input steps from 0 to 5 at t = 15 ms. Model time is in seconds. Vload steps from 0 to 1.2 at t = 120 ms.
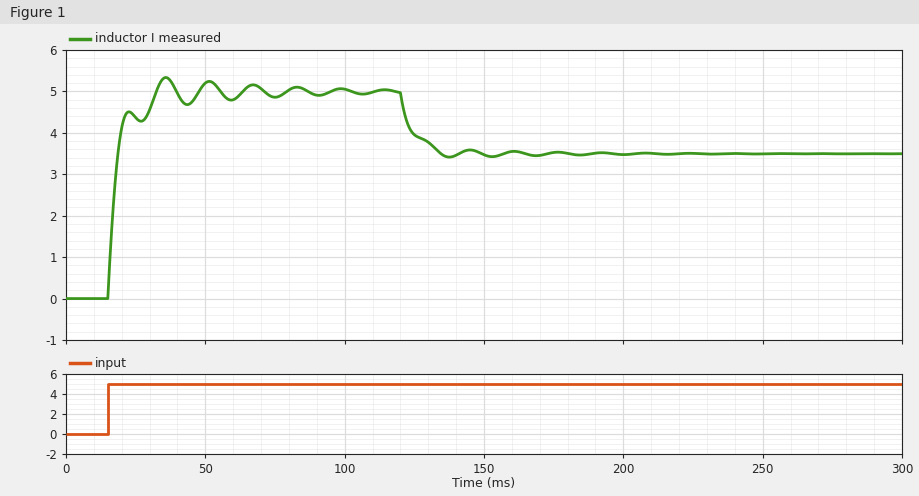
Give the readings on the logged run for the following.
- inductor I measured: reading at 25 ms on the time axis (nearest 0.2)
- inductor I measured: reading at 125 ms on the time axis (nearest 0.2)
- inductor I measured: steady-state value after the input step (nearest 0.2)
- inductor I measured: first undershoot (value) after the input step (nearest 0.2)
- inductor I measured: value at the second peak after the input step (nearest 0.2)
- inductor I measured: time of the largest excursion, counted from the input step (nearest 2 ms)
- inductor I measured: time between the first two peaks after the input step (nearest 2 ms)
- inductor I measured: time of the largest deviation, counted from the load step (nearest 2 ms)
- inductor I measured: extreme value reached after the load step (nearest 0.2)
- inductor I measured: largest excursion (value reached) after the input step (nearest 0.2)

4.4
4.0
5.0
4.6
5.2
20 ms
16 ms
18 ms
3.4
5.4
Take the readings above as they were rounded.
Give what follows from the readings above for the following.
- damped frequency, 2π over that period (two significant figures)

0.39 rad/ms
